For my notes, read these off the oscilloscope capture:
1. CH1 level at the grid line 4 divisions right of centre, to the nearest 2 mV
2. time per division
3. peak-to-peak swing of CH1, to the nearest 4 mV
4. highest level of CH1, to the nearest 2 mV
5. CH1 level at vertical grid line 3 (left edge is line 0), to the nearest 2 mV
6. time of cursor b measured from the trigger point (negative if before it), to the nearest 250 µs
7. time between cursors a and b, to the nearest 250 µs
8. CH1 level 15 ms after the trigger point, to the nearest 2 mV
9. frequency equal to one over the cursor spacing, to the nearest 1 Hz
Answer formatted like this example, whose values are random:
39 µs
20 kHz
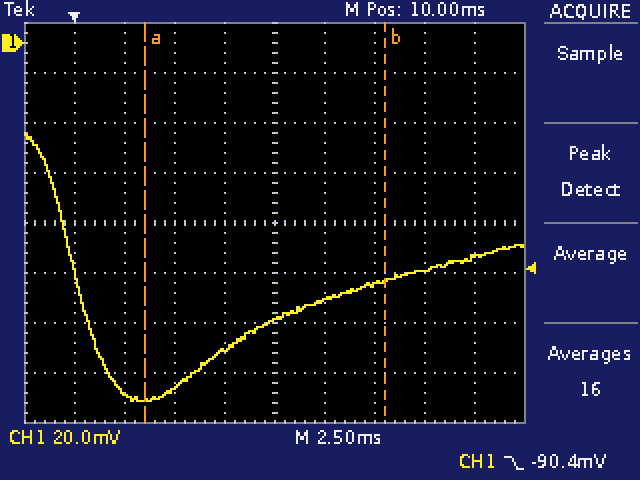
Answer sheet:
-86 mV
2.5 ms
108 mV
-36 mV
-138 mV
+15.50 ms
12.00 ms
-96 mV
83 Hz
